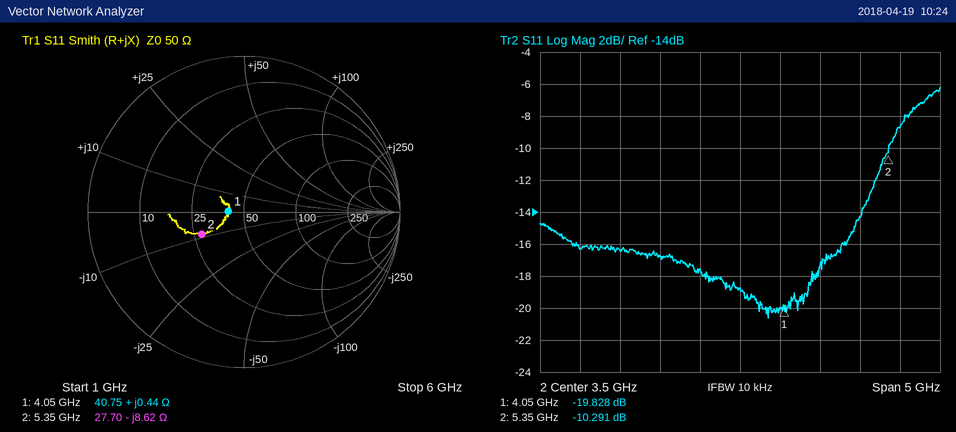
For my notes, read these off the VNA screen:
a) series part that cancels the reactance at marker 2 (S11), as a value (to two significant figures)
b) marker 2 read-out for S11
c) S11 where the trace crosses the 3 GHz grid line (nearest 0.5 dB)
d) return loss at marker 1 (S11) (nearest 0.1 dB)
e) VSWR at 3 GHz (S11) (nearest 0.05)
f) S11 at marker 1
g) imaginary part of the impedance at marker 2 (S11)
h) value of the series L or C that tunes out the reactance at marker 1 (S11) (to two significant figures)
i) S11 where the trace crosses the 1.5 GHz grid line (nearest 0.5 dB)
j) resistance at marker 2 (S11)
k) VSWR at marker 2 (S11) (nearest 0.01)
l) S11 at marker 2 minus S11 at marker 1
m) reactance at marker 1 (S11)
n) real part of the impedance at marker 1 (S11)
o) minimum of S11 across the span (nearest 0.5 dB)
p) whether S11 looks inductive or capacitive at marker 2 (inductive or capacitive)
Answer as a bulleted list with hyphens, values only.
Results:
- 260 pH
- -10.291 dB
- -17.5 dB
- 19.8 dB
- 1.30
- -19.828 dB
- -8.62 Ω
- 89 pF
- -16.5 dB
- 27.70 Ω
- 1.88
- 9.537 dB
- +0.44 Ω
- 40.75 Ω
- -20.5 dB
- capacitive
